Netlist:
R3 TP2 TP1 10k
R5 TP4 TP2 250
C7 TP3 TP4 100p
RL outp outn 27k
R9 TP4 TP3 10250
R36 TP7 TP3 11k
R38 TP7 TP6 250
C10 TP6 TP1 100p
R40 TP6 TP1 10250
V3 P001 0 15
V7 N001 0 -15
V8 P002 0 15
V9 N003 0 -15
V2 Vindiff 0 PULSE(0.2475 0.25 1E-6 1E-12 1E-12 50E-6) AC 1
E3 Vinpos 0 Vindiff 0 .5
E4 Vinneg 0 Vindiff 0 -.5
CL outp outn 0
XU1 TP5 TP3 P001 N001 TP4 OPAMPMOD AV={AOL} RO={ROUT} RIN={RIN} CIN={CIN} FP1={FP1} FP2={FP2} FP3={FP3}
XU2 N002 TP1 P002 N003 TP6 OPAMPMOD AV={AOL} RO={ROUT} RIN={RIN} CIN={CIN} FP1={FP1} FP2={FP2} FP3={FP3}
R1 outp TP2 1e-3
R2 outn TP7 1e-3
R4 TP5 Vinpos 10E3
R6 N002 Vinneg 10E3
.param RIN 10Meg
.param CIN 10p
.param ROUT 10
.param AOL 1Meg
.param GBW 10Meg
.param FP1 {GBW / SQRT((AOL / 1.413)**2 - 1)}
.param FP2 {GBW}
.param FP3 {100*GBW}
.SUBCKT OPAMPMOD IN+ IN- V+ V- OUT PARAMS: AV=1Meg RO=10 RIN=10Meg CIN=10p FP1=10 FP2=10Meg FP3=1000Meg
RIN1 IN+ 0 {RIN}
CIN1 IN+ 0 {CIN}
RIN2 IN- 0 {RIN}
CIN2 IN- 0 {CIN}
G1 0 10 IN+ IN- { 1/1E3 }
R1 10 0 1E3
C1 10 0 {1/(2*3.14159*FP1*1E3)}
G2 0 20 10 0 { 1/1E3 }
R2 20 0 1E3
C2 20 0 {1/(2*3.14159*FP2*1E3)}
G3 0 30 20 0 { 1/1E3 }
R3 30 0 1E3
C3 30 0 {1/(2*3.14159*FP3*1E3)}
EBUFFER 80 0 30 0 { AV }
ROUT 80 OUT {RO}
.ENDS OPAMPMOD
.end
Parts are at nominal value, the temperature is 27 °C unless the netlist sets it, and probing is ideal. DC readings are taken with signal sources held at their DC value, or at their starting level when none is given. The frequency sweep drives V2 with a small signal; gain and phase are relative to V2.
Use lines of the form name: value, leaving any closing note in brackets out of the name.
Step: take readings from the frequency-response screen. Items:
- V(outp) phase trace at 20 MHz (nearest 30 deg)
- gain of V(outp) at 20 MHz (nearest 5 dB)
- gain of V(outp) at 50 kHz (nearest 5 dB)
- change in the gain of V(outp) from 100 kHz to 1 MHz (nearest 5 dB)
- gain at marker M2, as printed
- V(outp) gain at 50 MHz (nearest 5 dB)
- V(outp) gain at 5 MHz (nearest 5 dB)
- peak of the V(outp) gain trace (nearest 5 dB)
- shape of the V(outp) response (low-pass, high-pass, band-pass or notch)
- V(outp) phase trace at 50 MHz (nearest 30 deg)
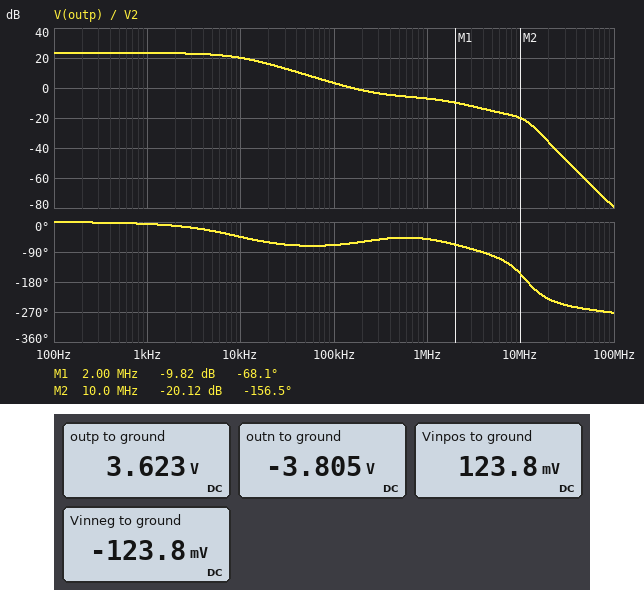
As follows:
V(outp) phase trace at 20 MHz: -240 deg
gain of V(outp) at 20 MHz: -35 dB
gain of V(outp) at 50 kHz: 10 dB
change in the gain of V(outp) from 100 kHz to 1 MHz: -10 dB
gain at marker M2, as printed: -20.12 dB
V(outp) gain at 50 MHz: -60 dB
V(outp) gain at 5 MHz: -15 dB
peak of the V(outp) gain trace: 25 dB
shape of the V(outp) response: low-pass
V(outp) phase trace at 50 MHz: -270 deg
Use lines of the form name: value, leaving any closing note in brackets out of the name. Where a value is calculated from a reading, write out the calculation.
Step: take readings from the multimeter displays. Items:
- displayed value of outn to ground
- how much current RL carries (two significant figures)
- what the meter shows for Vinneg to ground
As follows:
displayed value of outn to ground: -3.805 V
how much current RL carries: (3.623 V - (-3.805 V)) / 27 kΩ = 280 µA
what the meter shows for Vinneg to ground: -123.8 mV
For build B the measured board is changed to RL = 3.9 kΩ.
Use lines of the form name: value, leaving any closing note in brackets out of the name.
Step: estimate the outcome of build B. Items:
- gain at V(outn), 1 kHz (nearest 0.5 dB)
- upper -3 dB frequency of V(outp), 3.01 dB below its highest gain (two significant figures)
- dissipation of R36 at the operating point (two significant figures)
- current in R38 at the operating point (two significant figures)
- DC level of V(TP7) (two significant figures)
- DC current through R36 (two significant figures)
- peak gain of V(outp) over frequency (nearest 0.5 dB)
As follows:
gain at V(outn), 1 kHz: 15.0 dB
upper -3 dB frequency of V(outp), 3.01 dB below its highest gain: 23 kHz
dissipation of R36 at the operating point: 220 µW
current in R38 at the operating point: 850 µA
DC level of V(TP7): -1.4 V
DC current through R36: 140 µA
peak gain of V(outp) over frequency: 14.5 dB
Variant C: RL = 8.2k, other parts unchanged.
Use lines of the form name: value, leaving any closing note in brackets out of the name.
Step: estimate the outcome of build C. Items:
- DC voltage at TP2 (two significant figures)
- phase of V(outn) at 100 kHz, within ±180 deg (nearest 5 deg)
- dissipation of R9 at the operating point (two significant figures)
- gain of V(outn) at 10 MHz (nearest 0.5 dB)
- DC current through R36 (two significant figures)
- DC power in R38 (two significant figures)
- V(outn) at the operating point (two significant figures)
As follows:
DC voltage at TP2: 2.2 V
phase of V(outn) at 100 kHz, within ±180 deg: 115 deg
dissipation of R9 at the operating point: 500 µW
gain of V(outn) at 10 MHz: -20.5 dB
DC current through R36: 220 µA
DC power in R38: 150 µW
V(outn) at the operating point: -2.3 V
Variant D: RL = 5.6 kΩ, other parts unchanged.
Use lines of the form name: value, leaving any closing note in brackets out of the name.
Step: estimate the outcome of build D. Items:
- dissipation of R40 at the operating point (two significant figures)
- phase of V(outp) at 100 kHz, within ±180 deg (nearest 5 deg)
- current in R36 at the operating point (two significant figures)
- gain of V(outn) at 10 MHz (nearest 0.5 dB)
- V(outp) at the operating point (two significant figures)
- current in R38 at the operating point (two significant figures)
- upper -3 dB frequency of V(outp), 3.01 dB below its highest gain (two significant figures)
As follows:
dissipation of R40 at the operating point: 350 µW
phase of V(outp) at 100 kHz, within ±180 deg: -65 deg
current in R36 at the operating point: 180 µA
gain of V(outn) at 10 MHz: -20.5 dB
V(outp) at the operating point: 1.7 V
current in R38 at the operating point: 810 µA
upper -3 dB frequency of V(outp), 3.01 dB below its highest gain: 19 kHz
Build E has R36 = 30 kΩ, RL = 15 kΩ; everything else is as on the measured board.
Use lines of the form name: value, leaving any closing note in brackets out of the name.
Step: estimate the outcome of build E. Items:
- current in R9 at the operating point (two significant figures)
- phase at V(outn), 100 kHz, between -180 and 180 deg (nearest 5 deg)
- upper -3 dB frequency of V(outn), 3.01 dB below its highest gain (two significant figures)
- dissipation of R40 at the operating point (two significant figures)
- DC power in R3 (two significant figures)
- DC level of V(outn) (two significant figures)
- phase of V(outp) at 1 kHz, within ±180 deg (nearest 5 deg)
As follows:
current in R9 at the operating point: 23 µA
phase at V(outn), 100 kHz, between -180 and 180 deg: 140 deg
upper -3 dB frequency of V(outn), 3.01 dB below its highest gain: 74 kHz
dissipation of R40 at the operating point: 22 µW
DC power in R3: 21 µW
DC level of V(outn): -570 mV
phase of V(outp) at 1 kHz, within ±180 deg: 0 deg
